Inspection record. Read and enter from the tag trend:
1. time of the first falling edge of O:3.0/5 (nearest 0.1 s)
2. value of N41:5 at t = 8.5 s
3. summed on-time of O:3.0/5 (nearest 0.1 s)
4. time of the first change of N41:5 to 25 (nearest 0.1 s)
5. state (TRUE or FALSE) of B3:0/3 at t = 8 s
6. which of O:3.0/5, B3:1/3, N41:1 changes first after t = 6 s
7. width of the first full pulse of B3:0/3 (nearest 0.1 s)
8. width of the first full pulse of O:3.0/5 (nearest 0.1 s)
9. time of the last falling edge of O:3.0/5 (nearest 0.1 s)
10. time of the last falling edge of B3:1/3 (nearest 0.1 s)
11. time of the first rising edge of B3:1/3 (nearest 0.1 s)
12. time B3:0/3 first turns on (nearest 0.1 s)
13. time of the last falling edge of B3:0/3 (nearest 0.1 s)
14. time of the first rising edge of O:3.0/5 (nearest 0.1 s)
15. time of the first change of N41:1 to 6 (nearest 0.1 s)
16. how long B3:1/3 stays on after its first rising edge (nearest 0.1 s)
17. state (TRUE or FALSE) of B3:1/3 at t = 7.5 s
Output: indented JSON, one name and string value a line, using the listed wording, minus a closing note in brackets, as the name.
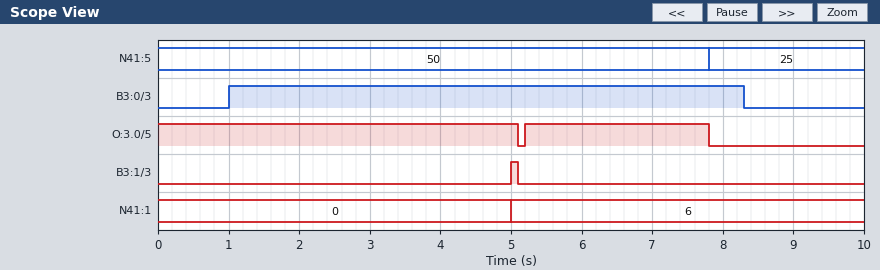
{
  "time of the first falling edge of O:3.0/5": "5.1 s",
  "value of N41:5 at t = 8.5 s": "25",
  "summed on-time of O:3.0/5": "7.7 s",
  "time of the first change of N41:5 to 25": "7.8 s",
  "state (TRUE or FALSE) of B3:0/3 at t = 8 s": "TRUE",
  "which of O:3.0/5, B3:1/3, N41:1 changes first after t = 6 s": "O:3.0/5",
  "width of the first full pulse of B3:0/3": "7.3 s",
  "width of the first full pulse of O:3.0/5": "2.6 s",
  "time of the last falling edge of O:3.0/5": "7.8 s",
  "time of the last falling edge of B3:1/3": "5.1 s",
  "time of the first rising edge of B3:1/3": "5.0 s",
  "time B3:0/3 first turns on": "1.0 s",
  "time of the last falling edge of B3:0/3": "8.3 s",
  "time of the first rising edge of O:3.0/5": "5.2 s",
  "time of the first change of N41:1 to 6": "5.0 s",
  "how long B3:1/3 stays on after its first rising edge": "0.1 s",
  "state (TRUE or FALSE) of B3:1/3 at t = 7.5 s": "FALSE"
}
